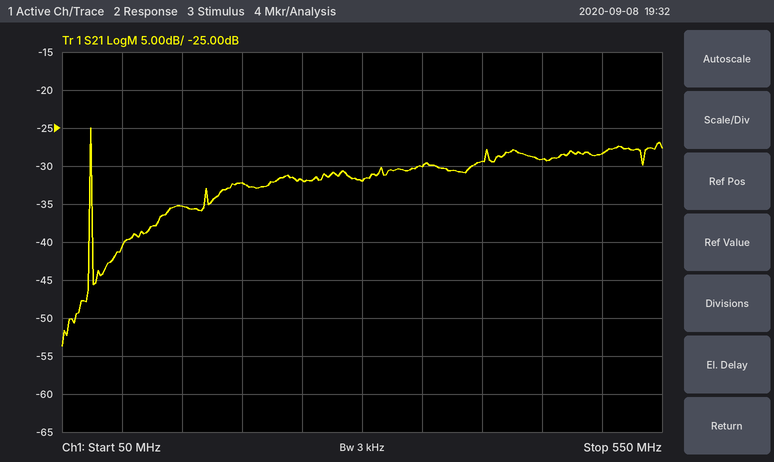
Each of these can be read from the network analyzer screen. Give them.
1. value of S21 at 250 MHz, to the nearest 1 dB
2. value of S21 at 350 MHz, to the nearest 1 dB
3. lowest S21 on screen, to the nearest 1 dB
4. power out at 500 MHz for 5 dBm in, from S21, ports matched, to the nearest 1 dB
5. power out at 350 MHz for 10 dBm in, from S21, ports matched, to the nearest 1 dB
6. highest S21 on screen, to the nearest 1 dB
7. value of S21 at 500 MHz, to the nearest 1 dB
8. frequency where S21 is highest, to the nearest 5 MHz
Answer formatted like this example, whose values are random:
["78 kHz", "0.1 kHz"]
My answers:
["-32 dB", "-30 dB", "-54 dB", "-23 dBm", "-20 dBm", "-25 dB", "-28 dB", "75 MHz"]
